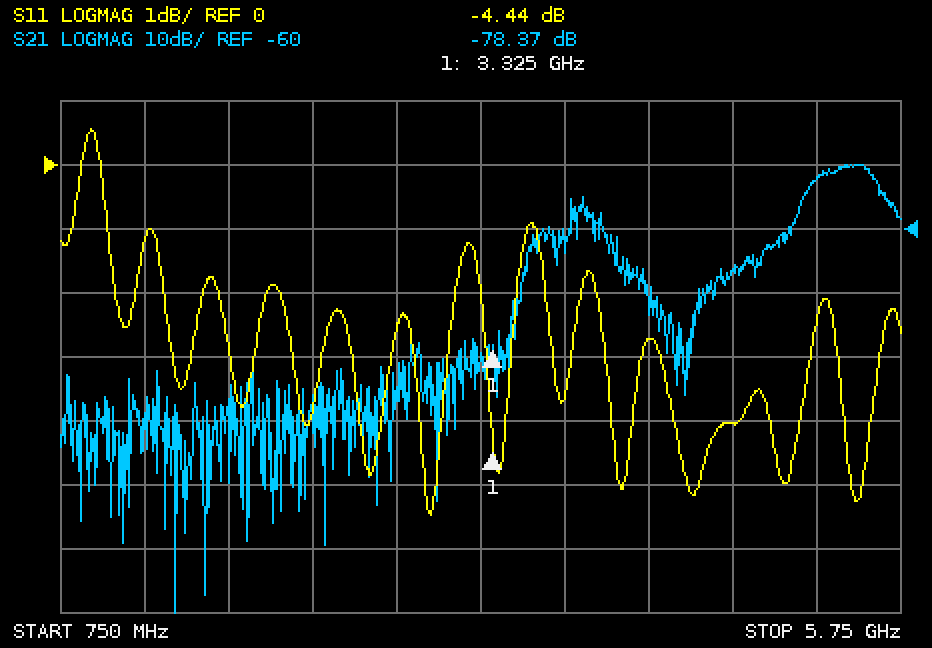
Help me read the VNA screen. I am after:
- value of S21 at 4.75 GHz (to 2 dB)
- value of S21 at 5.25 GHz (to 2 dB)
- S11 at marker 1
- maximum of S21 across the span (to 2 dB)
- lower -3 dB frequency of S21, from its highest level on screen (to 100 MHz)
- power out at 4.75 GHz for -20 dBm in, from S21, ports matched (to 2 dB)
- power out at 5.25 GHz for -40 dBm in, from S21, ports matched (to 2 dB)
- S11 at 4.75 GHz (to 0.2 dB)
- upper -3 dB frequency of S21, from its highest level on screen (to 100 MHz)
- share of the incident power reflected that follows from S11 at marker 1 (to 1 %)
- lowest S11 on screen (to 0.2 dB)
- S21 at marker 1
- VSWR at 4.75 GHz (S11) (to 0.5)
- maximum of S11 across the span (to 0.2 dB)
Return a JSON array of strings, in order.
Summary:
["-66 dB", "-52 dB", "-4.44 dB", "-50 dB", "5.2 GHz", "-86 dBm", "-92 dBm", "-4.0 dB", "5.6 GHz", "36 %", "-5.4 dB", "-78.37 dB", "4.5", "0.6 dB"]
